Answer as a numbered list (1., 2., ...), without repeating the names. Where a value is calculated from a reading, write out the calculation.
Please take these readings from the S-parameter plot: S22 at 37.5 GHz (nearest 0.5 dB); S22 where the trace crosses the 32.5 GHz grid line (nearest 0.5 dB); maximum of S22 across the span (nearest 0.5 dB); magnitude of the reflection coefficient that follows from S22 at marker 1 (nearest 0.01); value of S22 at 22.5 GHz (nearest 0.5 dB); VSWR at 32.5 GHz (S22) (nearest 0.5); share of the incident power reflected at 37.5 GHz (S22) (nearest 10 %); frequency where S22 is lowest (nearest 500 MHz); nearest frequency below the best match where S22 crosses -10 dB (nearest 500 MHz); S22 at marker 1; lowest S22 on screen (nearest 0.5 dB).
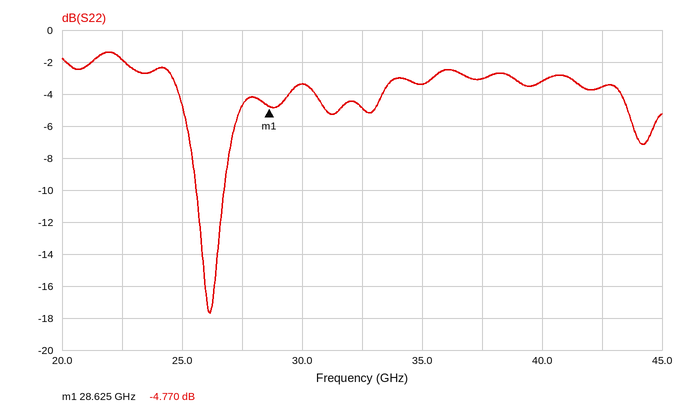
1. -3.0 dB
2. -5.0 dB
3. -1.5 dB
4. 10^(-4.77/20) ≈ 0.58
5. -2.0 dB
6. |Γ| = 10^(-5/20) = 0.5623; VSWR = (1 + 0.5623)/(1 − 0.5623) ≈ 3.57, so 3.5 to the nearest 0.5
7. 10^(-3/10) ≈ 50 %
8. 26.0 GHz
9. 25.5 GHz
10. -4.770 dB
11. -17.5 dB
